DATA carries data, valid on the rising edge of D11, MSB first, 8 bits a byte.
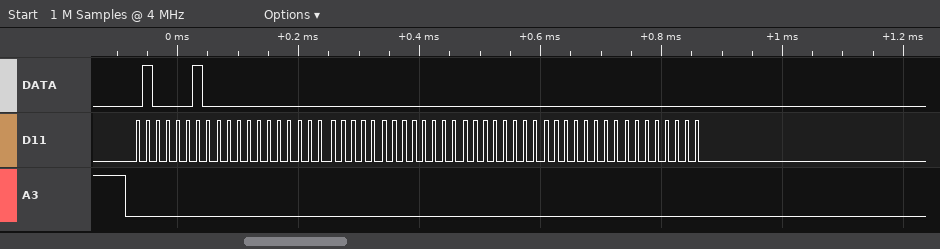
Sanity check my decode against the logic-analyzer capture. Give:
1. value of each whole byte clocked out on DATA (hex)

0x42 0x00 0x00 0x00 0x00 0x00 0x00
